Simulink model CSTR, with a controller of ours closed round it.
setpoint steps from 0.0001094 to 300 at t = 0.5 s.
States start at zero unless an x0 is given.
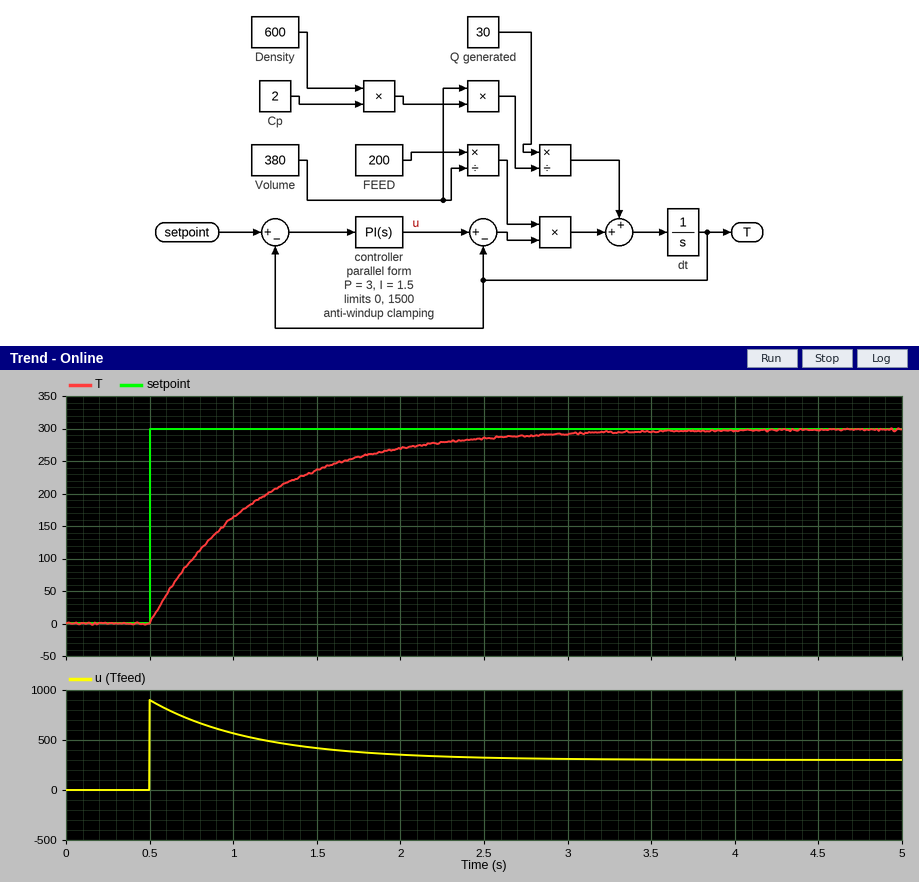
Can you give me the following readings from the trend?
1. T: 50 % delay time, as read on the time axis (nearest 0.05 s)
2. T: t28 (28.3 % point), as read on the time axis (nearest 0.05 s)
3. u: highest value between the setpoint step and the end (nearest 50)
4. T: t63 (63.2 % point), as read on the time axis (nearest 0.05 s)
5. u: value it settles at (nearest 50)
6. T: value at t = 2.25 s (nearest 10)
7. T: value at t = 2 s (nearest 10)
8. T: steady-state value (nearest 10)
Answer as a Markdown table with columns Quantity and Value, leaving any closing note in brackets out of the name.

| Quantity | Value |
|---|---|
| T: 50 % delay time, as read on the time axis | 0.95 s |
| T: t28 (28.3 % point), as read on the time axis | 0.70 s |
| u: highest value between the setpoint step and the end | 900 |
| T: t63 (63.2 % point), as read on the time axis | 1.15 s |
| u: value it settles at | 300 |
| T: value at t = 2.25 s | 280 |
| T: value at t = 2 s | 270 |
| T: steady-state value | 300 |
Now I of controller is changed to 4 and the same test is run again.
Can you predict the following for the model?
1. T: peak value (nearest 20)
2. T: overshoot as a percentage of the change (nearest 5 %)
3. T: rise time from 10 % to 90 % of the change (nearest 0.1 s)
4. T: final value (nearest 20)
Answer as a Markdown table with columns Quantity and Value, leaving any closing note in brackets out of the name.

| Quantity | Value |
|---|---|
| T: peak value | 340 |
| T: overshoot as a percentage of the change | 10 % |
| T: rise time from 10 % to 90 % of the change | 0.8 s |
| T: final value | 300 |
